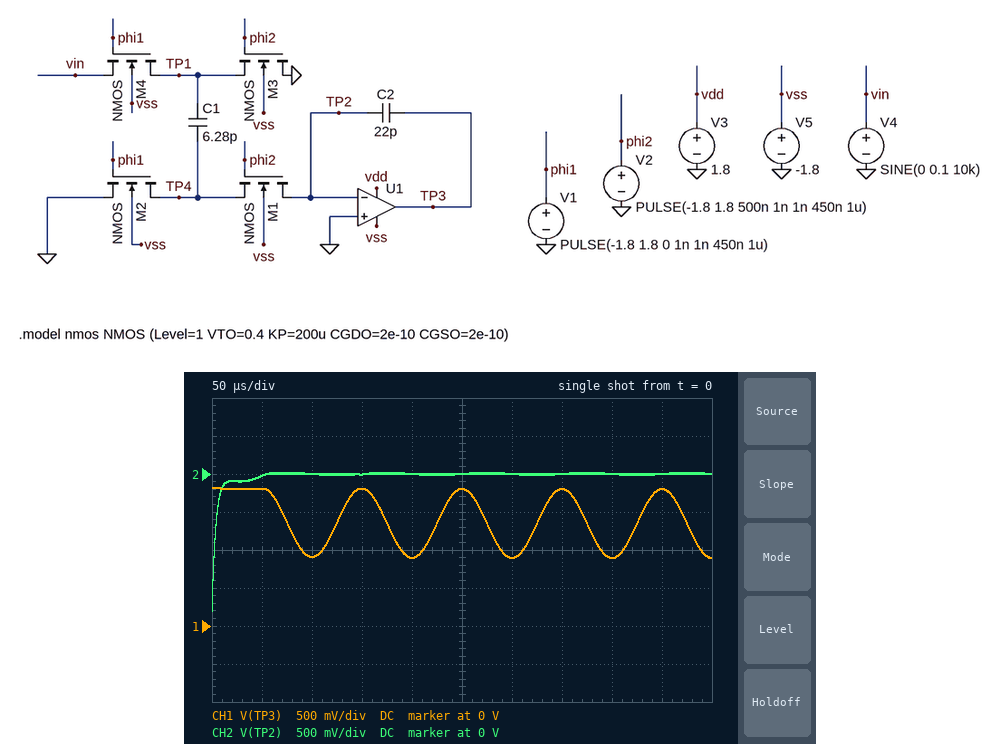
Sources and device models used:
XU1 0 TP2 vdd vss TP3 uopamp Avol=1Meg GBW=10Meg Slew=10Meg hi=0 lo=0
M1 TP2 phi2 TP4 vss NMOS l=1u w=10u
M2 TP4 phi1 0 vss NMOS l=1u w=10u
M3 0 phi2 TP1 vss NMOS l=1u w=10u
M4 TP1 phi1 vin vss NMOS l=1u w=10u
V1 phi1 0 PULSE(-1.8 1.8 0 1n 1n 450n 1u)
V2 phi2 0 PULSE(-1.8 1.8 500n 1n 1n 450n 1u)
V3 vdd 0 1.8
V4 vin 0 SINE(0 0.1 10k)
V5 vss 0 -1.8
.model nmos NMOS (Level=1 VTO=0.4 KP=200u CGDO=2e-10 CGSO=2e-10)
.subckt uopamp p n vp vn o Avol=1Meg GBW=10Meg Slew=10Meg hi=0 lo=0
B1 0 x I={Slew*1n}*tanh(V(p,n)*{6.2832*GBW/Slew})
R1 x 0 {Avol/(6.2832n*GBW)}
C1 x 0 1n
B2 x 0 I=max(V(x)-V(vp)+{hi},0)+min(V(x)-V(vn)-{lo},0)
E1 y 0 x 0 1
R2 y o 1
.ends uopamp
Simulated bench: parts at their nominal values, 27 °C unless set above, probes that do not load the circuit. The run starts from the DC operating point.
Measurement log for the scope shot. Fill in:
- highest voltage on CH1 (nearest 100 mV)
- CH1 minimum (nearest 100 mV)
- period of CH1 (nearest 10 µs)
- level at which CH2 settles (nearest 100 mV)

1.8 V
900 mV
100 µs
0 V
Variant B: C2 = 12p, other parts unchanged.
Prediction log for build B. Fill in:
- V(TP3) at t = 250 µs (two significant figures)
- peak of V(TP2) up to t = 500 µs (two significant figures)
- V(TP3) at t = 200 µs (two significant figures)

1.8 V
25 mV
140 mV
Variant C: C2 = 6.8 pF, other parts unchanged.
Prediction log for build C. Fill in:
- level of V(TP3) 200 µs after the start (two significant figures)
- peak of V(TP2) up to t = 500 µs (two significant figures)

-1.1 V
38 mV
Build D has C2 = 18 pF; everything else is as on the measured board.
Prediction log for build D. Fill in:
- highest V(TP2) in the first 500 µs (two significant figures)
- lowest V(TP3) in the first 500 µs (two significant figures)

18 mV
690 mV
